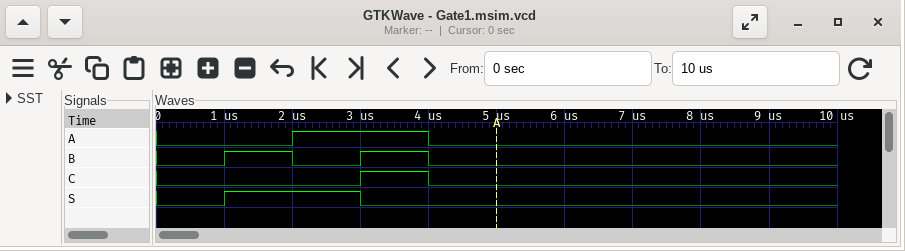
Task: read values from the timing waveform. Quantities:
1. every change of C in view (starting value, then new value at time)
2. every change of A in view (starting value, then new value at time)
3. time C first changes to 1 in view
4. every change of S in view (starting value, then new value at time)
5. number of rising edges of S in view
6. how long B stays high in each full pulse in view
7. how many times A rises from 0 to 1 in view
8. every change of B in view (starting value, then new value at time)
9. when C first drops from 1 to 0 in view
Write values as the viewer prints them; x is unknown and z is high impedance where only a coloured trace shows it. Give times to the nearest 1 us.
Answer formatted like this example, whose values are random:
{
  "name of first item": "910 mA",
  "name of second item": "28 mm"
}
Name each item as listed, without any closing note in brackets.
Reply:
{
  "every change of C in view": "0, 1 at 3 us, 0 at 4 us",
  "every change of A in view": "0, 1 at 2 us, 0 at 4 us",
  "time C first changes to 1 in view": "3 us",
  "every change of S in view": "0, 1 at 1 us, 0 at 3 us",
  "number of rising edges of S in view": "1",
  "how long B stays high in each full pulse in view": "1 us, 1 us",
  "how many times A rises from 0 to 1 in view": "1",
  "every change of B in view": "0, 1 at 1 us, 0 at 2 us, 1 at 3 us, 0 at 4 us",
  "when C first drops from 1 to 0 in view": "4 us"
}
